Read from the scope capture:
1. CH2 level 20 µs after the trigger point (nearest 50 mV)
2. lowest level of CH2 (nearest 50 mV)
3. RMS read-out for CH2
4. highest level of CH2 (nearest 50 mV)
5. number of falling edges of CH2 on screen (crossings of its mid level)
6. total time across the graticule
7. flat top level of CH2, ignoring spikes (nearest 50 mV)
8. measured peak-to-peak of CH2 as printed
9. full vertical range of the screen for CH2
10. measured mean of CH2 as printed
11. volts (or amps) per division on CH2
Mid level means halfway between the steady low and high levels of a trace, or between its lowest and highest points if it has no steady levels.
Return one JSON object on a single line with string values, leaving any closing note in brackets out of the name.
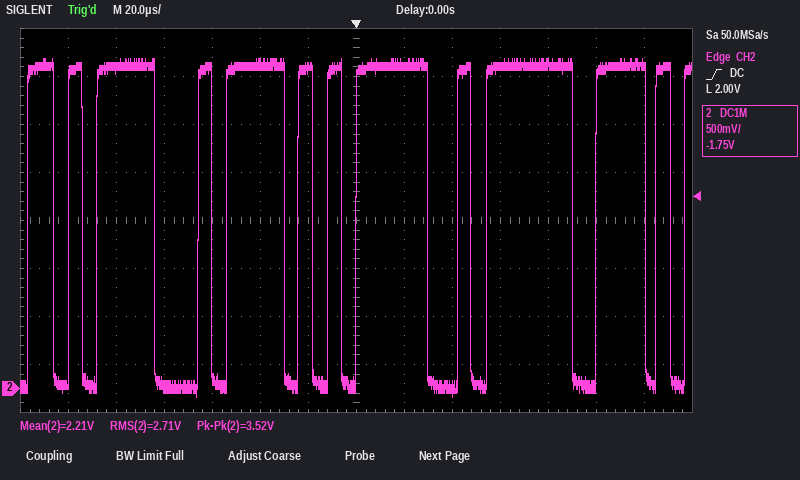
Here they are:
{"CH2 level 20 µs after the trigger point": "3.35 V", "lowest level of CH2": "-100 mV", "RMS read-out for CH2": "2.71 V", "highest level of CH2": "3.45 V", "number of falling edges of CH2 on screen": "12", "total time across the graticule": "280 µs", "flat top level of CH2, ignoring spikes": "3.35 V", "measured peak-to-peak of CH2 as printed": "3.52 V", "full vertical range of the screen for CH2": "4 V", "measured mean of CH2 as printed": "2.21 V", "volts (or amps) per division on CH2": "500 mV"}
